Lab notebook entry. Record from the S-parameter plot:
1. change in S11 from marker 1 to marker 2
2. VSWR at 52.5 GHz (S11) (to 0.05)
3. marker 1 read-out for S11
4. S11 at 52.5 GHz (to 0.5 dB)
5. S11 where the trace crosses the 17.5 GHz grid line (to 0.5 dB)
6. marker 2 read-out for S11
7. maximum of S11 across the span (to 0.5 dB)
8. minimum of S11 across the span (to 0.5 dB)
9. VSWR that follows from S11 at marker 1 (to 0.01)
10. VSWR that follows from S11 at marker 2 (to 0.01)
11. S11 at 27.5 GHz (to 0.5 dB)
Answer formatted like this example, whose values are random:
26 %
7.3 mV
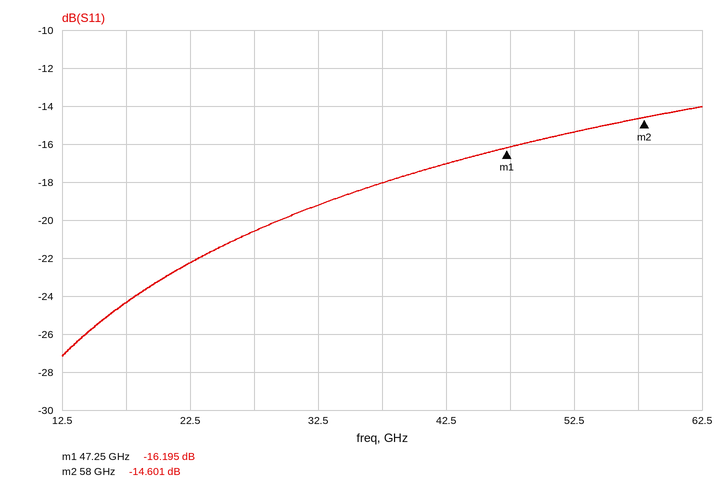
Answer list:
1.594 dB
1.40
-16.195 dB
-15.5 dB
-24.5 dB
-14.601 dB
-14.0 dB
-27.0 dB
1.37
1.46
-20.5 dB
